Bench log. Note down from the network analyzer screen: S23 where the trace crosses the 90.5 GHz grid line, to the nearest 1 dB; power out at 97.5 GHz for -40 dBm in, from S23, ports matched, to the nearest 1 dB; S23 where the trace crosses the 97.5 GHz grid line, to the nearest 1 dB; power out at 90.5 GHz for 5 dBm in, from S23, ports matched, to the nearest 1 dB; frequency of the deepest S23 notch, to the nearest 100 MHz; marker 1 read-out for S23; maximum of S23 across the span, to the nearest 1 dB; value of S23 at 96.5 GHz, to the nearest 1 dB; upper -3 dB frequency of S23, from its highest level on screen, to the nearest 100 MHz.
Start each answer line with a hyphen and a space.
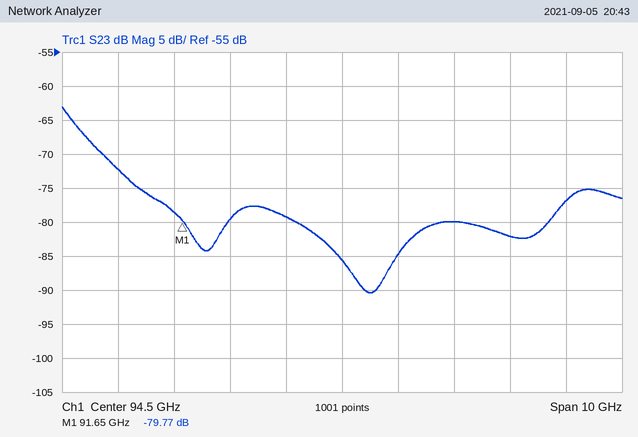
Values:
- -72 dB
- -122 dBm
- -82 dB
- -67 dBm
- 95.0 GHz
- -79.77 dB
- -63 dB
- -80 dB
- 89.8 GHz
